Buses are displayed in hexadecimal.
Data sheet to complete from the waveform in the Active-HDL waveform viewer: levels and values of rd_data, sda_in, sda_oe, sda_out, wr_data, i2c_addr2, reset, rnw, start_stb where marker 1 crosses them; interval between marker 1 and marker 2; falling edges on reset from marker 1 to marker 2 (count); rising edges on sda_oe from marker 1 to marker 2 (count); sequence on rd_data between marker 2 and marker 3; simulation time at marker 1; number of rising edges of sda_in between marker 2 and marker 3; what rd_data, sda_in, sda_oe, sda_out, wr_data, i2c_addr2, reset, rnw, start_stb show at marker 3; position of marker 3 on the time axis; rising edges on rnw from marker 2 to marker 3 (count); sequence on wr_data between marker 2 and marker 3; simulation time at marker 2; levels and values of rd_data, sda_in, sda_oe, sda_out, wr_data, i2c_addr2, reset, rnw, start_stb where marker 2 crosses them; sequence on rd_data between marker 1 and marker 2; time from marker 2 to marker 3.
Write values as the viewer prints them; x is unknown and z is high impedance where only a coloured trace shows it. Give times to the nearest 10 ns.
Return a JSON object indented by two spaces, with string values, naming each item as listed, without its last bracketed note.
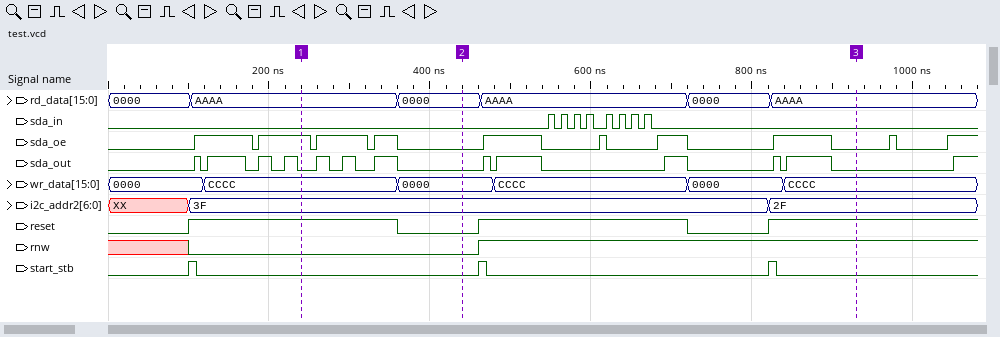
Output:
{
  "levels and values of rd_data, sda_in, sda_oe, sda_out, wr_data, i2c_addr2, reset, rnw, start_stb where marker 1 crosses them": "rd_data=AAAA, sda_in=0, sda_oe=1, sda_out=0, wr_data=CCCC, i2c_addr2=3F, reset=1, rnw=0, start_stb=0",
  "interval between marker 1 and marker 2": "200 ns",
  "falling edges on reset from marker 1 to marker 2": "1",
  "rising edges on sda_oe from marker 1 to marker 2": "2",
  "sequence on rd_data between marker 2 and marker 3": "0000, AAAA, 0000, AAAA",
  "simulation time at marker 1": "240 ns",
  "number of rising edges of sda_in between marker 2 and marker 3": "8",
  "what rd_data, sda_in, sda_oe, sda_out, wr_data, i2c_addr2, reset, rnw, start_stb show at marker 3": "rd_data=AAAA, sda_in=0, sda_oe=0, sda_out=0, wr_data=CCCC, i2c_addr2=2F, reset=1, rnw=1, start_stb=0",
  "position of marker 3 on the time axis": "930 ns",
  "rising edges on rnw from marker 2 to marker 3": "1",
  "sequence on wr_data between marker 2 and marker 3": "0000, CCCC, 0000, CCCC",
  "simulation time at marker 2": "440 ns",
  "levels and values of rd_data, sda_in, sda_oe, sda_out, wr_data, i2c_addr2, reset, rnw, start_stb where marker 2 crosses them": "rd_data=0000, sda_in=0, sda_oe=0, sda_out=0, wr_data=0000, i2c_addr2=3F, reset=0, rnw=0, start_stb=0",
  "sequence on rd_data between marker 1 and marker 2": "AAAA, 0000",
  "time from marker 2 to marker 3": "490 ns"
}
